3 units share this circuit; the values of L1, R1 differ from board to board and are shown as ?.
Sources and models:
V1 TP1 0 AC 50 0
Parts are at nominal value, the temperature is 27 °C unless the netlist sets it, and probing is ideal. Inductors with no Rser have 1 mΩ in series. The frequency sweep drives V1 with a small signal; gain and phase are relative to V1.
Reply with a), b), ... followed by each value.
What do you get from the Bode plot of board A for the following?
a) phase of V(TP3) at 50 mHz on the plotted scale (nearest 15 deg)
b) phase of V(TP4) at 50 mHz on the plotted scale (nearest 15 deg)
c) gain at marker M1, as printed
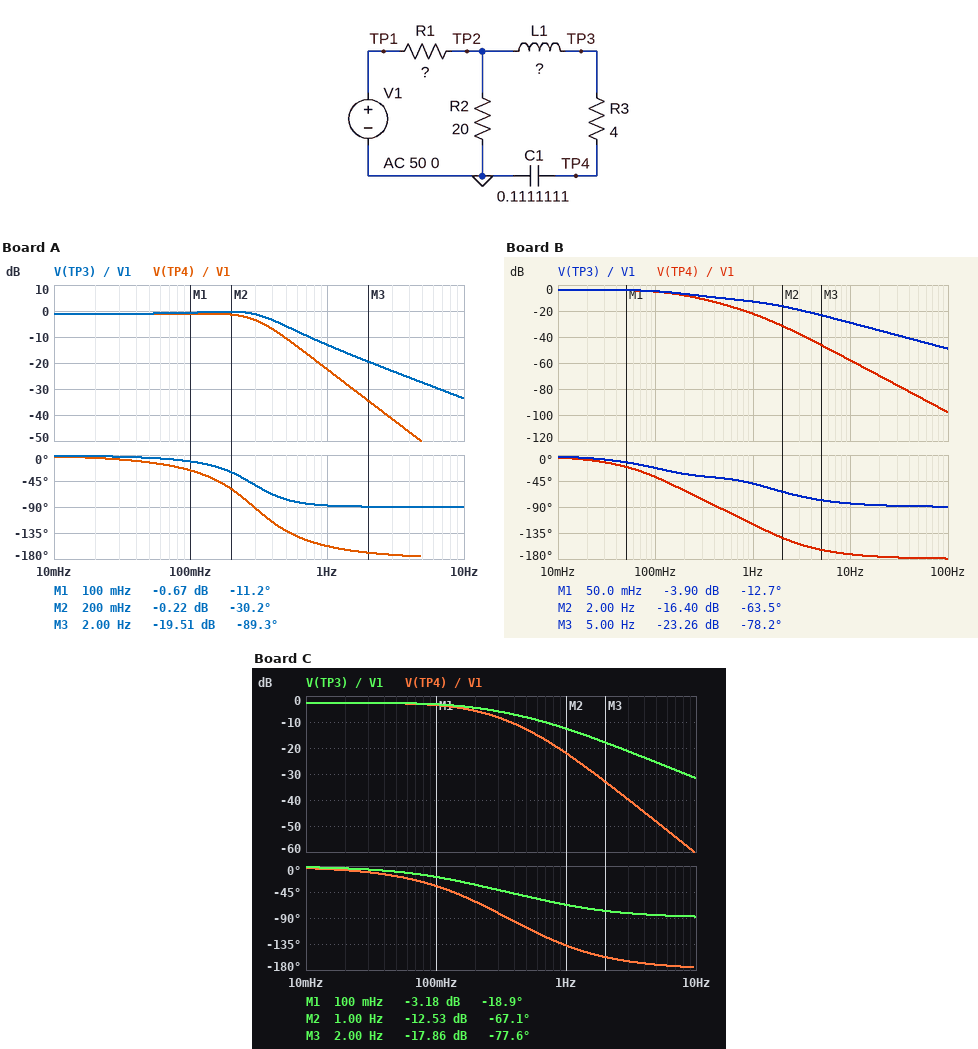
a) 0 deg
b) -15 deg
c) -0.67 dB
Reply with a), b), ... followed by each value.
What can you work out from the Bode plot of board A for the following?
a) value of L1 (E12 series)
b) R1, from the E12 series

a) 2.7 H
b) 2.7 Ω
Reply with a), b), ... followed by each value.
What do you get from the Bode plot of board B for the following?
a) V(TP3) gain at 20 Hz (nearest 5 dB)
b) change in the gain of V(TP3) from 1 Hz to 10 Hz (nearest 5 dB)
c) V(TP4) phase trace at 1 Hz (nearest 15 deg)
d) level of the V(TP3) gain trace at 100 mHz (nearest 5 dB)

a) -35 dB
b) -15 dB
c) -120 deg
d) -5 dB
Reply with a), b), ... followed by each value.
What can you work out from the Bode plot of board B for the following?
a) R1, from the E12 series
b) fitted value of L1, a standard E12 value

a) 10 Ω
b) 1.2 H
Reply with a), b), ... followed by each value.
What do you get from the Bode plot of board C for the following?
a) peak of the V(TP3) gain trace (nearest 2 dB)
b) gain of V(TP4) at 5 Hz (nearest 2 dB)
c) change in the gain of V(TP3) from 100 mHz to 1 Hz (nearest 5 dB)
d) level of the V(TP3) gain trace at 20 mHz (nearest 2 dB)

a) -2 dB
b) -48 dB
c) -10 dB
d) -2 dB
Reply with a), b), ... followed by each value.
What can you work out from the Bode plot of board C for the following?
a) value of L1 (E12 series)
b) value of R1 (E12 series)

a) 1.8 H
b) 6.8 Ω
